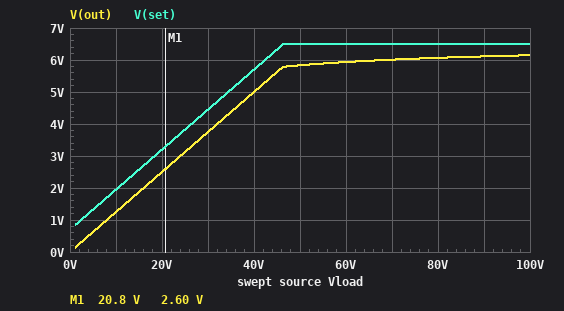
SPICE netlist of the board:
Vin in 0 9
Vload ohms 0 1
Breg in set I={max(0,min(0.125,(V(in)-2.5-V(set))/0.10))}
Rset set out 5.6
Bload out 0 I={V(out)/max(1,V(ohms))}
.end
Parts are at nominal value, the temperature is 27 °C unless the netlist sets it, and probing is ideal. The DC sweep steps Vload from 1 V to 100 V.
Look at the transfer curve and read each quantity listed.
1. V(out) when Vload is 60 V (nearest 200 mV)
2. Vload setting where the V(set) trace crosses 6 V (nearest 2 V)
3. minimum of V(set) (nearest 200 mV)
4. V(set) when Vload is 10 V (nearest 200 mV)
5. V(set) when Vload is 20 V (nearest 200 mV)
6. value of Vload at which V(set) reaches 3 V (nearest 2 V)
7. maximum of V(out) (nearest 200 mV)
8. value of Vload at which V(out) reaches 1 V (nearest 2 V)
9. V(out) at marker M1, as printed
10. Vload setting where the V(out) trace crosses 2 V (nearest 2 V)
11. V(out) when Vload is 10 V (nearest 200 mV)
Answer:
6.0 V
42 V
800 mV
2.0 V
3.2 V
18 V
6.2 V
8 V
2.60 V
16 V
1.2 V
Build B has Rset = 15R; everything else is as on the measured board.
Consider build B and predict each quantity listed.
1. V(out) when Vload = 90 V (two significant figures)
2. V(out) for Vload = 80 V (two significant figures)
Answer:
5.6 V
5.5 V
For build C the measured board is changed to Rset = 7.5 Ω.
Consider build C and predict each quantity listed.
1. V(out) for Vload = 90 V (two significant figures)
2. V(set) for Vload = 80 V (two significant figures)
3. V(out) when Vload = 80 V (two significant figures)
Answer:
6.0 V
6.5 V
5.9 V
